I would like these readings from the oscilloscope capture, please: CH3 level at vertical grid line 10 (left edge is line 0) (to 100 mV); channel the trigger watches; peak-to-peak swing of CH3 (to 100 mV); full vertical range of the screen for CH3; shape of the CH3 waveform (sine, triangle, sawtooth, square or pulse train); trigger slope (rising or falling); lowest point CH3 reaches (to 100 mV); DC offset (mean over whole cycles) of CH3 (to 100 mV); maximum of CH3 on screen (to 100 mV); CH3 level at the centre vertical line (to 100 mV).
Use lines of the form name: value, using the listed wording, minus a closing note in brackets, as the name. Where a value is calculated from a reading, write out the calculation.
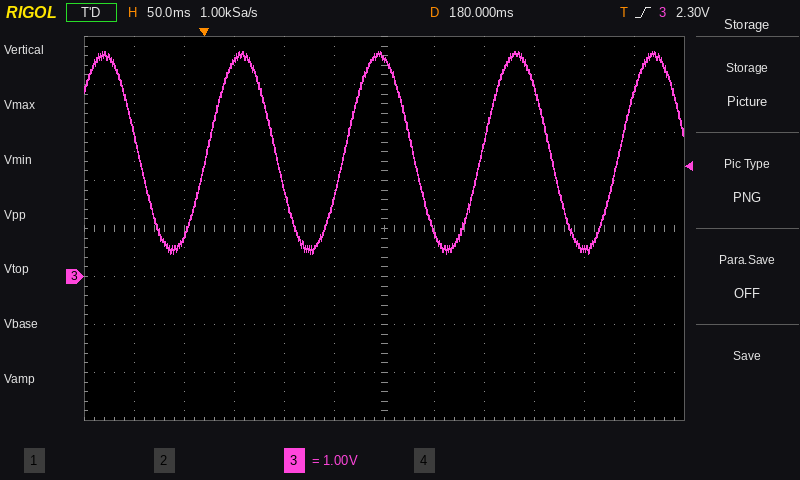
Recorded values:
CH3 level at vertical grid line 10 (left edge is line 0): 600 mV
channel the trigger watches: CH3
peak-to-peak swing of CH3: 4.7 V − (500 mV) = 4.2 V
full vertical range of the screen for CH3: 8 V
shape of the CH3 waveform: sine
trigger slope: rising
lowest point CH3 reaches: 500 mV
DC offset (mean over whole cycles) of CH3: (4.7 V + (500 mV)) / 2 ≈ 2.6 V
maximum of CH3 on screen: 4.7 V
CH3 level at the centre vertical line: 4.6 V
